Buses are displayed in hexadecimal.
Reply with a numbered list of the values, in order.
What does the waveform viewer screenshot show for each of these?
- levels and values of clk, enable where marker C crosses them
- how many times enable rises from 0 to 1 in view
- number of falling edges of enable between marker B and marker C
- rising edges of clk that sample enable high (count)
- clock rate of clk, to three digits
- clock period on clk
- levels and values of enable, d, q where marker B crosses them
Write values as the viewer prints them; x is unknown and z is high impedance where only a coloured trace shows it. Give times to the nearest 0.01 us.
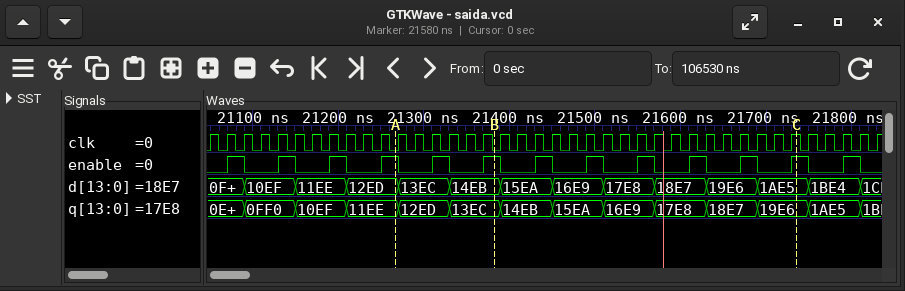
1. clk=1, enable=1
2. 13
3. 6
4. 13
5. 50.0 MHz
6. 0.02 us
7. enable=1, d=14EB, q=13EC
